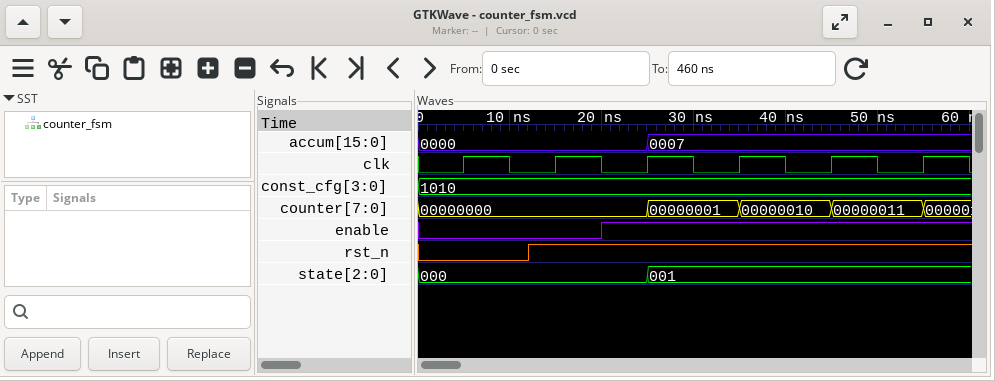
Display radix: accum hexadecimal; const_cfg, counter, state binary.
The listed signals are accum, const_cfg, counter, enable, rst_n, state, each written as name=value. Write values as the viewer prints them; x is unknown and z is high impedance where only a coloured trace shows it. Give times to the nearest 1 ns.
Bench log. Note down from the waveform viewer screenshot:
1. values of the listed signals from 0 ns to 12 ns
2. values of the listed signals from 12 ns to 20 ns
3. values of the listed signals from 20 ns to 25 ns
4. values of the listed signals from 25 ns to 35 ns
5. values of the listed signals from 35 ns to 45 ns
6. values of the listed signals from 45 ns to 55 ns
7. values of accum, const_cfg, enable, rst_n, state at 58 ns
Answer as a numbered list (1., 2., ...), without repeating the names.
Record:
1. accum=0000, const_cfg=1010, counter=00000000, enable=0, rst_n=0, state=000
2. accum=0000, const_cfg=1010, counter=00000000, enable=0, rst_n=1, state=000
3. accum=0000, const_cfg=1010, counter=00000000, enable=1, rst_n=1, state=000
4. accum=0007, const_cfg=1010, counter=00000001, enable=1, rst_n=1, state=001
5. accum=0007, const_cfg=1010, counter=00000010, enable=1, rst_n=1, state=001
6. accum=0007, const_cfg=1010, counter=00000011, enable=1, rst_n=1, state=001
7. accum=0007, const_cfg=1010, enable=1, rst_n=1, state=001
